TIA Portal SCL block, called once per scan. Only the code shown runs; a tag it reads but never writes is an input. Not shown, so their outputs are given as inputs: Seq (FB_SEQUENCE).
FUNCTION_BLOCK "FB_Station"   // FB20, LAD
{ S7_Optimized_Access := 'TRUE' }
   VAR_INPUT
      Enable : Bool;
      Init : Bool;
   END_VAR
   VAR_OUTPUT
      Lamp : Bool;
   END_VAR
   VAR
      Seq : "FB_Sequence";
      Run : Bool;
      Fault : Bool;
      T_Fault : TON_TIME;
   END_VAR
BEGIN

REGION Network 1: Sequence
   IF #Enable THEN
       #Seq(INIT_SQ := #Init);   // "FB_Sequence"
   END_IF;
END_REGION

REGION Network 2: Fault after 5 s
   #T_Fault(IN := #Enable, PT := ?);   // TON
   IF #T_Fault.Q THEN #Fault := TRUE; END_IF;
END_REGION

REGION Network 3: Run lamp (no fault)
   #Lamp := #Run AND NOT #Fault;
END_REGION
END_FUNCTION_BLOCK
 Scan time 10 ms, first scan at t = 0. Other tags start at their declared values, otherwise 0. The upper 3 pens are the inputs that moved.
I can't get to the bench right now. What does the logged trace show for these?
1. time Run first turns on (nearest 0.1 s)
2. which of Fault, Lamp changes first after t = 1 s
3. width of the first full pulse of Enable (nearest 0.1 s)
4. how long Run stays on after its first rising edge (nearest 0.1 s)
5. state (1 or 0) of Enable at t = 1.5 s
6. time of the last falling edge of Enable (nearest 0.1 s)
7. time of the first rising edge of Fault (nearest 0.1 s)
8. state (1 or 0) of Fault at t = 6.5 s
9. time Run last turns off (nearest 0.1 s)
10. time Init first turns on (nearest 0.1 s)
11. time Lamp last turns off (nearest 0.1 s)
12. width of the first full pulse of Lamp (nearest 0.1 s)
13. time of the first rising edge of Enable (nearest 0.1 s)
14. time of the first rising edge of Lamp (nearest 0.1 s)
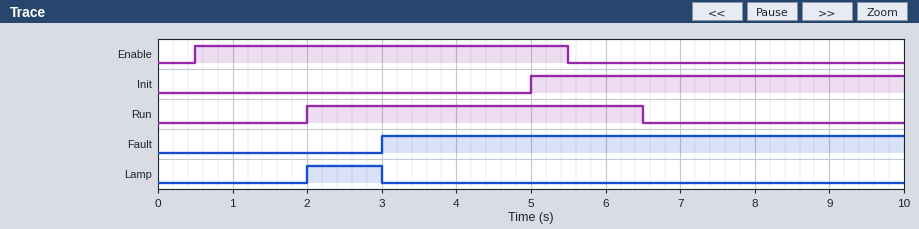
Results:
2.0 s
Lamp
5.0 s
4.5 s
1
5.5 s
3.0 s
1
6.5 s
5.0 s
3.0 s
1.0 s
0.5 s
2.0 s
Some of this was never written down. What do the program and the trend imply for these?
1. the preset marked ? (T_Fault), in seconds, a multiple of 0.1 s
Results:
2.5 s
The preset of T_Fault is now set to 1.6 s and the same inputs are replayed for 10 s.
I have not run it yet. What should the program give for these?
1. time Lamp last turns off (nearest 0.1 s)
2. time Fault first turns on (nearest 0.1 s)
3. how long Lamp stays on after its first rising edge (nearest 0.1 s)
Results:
2.1 s
2.1 s
0.1 s
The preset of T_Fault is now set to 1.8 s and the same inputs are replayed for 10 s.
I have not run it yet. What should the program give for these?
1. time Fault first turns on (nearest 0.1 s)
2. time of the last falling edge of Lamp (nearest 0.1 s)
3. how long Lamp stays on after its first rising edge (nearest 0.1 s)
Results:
2.3 s
2.3 s
0.3 s
